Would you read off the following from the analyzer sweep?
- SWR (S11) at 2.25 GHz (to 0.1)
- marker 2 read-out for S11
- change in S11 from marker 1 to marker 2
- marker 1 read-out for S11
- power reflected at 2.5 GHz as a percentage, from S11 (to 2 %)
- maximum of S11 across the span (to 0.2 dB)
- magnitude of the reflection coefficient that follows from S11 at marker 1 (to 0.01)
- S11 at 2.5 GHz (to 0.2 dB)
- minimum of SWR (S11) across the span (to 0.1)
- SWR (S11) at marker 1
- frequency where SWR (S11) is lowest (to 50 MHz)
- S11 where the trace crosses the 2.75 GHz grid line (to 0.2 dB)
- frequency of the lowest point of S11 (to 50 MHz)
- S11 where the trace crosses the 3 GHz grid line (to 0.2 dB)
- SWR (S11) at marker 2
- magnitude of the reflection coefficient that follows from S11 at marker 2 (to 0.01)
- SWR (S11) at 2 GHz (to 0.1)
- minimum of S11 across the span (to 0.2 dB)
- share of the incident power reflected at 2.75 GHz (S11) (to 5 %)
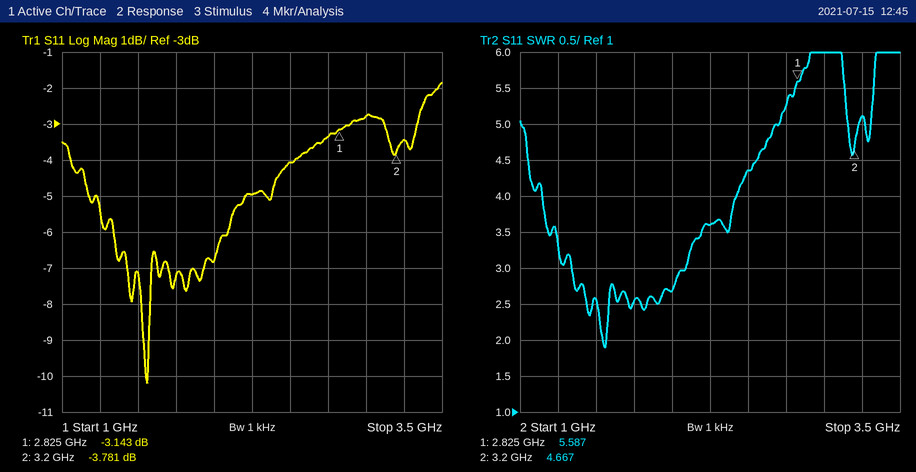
3.6
-3.781 dB
-0.638 dB
-3.143 dB
40 %
-1.8 dB
0.70
-4.0 dB
1.9
5.587
1.55 GHz
-3.4 dB
1.55 GHz
-2.8 dB
4.667
0.65
2.7
-10.2 dB
45 %
